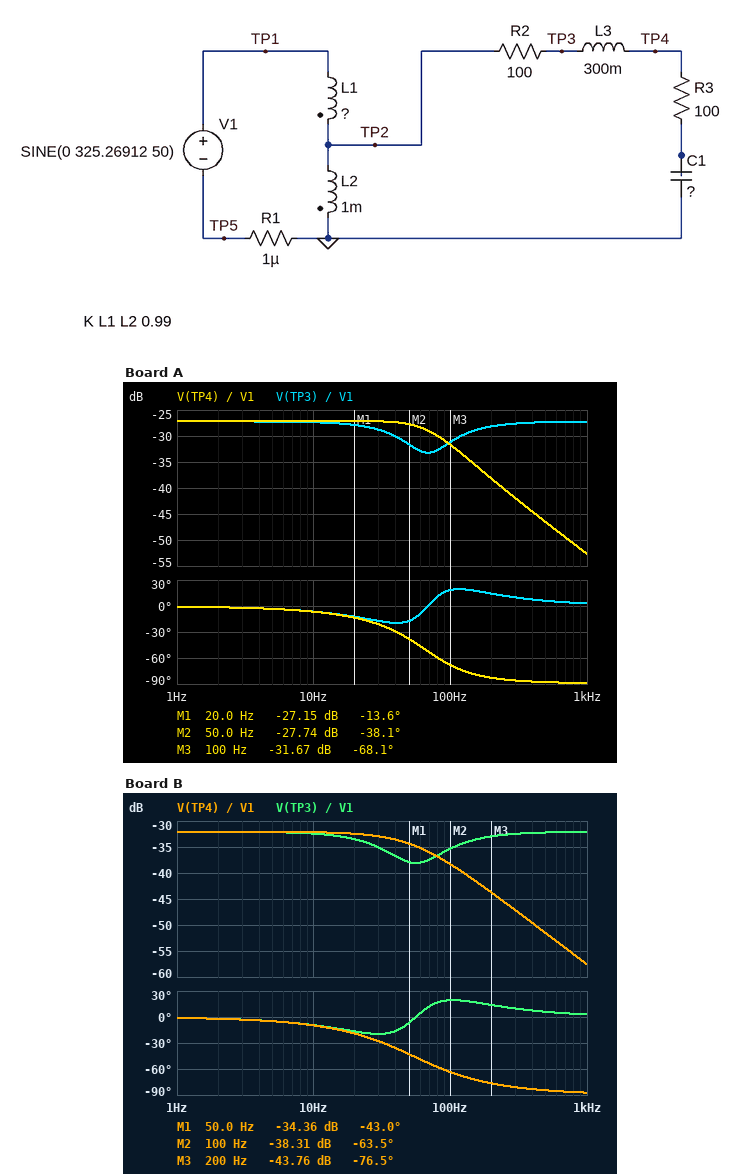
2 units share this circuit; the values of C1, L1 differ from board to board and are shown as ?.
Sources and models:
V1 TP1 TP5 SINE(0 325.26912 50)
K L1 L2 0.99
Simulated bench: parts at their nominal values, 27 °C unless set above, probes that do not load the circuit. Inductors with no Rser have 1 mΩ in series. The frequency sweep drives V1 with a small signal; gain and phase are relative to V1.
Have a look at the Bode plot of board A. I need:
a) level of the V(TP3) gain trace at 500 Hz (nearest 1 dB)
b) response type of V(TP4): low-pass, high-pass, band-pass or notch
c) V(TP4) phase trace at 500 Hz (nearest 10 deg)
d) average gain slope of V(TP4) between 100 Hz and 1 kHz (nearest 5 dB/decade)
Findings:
-27 dB
low-pass
-90 deg
-20 dB/decade
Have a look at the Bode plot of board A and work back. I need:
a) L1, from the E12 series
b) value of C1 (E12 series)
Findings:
470 mH
18 µF
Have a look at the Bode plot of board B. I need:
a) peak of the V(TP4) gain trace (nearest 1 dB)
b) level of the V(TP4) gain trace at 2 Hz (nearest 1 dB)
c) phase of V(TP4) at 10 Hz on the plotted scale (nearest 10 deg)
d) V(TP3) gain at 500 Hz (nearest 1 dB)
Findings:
-32 dB
-32 dB
-10 deg
-32 dB
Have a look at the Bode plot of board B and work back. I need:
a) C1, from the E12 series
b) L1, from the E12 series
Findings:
27 µF
1.5 H
